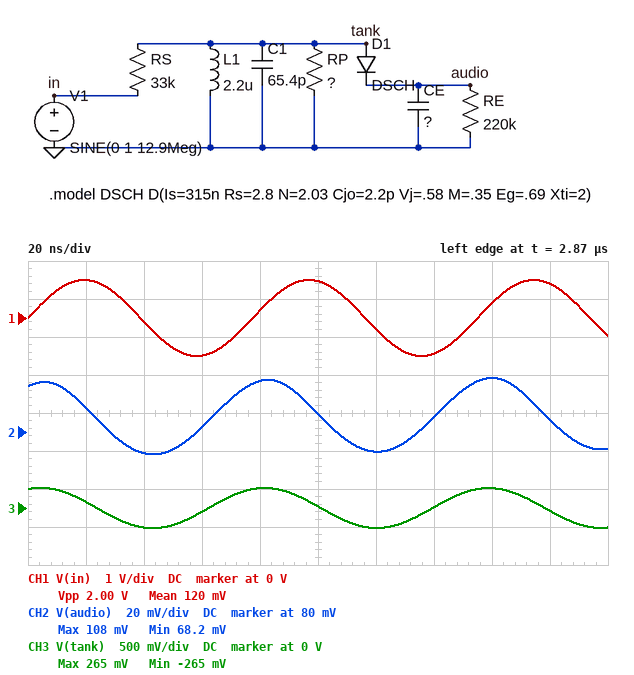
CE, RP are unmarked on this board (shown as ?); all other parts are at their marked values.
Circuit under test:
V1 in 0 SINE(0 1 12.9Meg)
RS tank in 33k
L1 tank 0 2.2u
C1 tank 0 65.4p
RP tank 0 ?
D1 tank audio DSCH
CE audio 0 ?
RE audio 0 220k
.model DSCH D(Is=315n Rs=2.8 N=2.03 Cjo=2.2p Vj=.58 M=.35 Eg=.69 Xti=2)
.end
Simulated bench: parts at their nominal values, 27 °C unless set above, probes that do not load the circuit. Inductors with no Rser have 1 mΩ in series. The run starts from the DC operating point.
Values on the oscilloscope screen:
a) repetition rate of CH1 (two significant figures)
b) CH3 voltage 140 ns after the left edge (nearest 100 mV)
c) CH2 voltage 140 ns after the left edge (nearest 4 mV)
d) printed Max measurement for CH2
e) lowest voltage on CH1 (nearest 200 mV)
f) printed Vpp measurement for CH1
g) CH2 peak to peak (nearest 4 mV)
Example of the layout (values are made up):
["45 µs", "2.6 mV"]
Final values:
["13 MHz", "0 V", "88 mV", "108 mV", "-1.0 V", "2.00 V", "40 mV"]
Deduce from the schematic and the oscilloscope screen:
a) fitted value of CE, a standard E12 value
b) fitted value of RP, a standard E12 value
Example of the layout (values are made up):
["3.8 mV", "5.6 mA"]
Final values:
["27 pF", "100 kΩ"]
